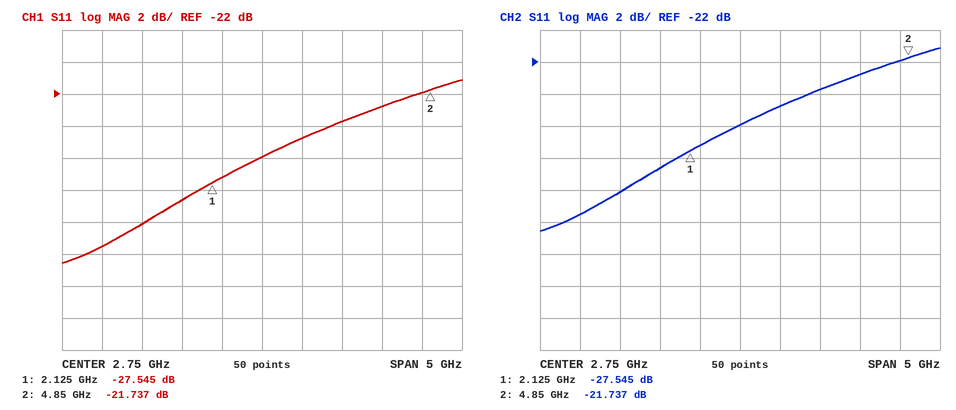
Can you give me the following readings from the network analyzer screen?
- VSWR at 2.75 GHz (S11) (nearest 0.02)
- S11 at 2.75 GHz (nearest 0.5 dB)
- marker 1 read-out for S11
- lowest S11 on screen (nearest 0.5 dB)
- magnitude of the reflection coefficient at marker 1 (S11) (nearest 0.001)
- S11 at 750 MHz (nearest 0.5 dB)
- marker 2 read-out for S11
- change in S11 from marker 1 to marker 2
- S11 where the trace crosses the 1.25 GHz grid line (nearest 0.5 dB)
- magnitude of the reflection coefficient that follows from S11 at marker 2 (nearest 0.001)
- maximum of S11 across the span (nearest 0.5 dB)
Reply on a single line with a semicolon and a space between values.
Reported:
1.10; -26.0 dB; -27.545 dB; -32.5 dB; 0.042; -31.5 dB; -21.737 dB; 5.808 dB; -30.0 dB; 0.082; -21.0 dB
